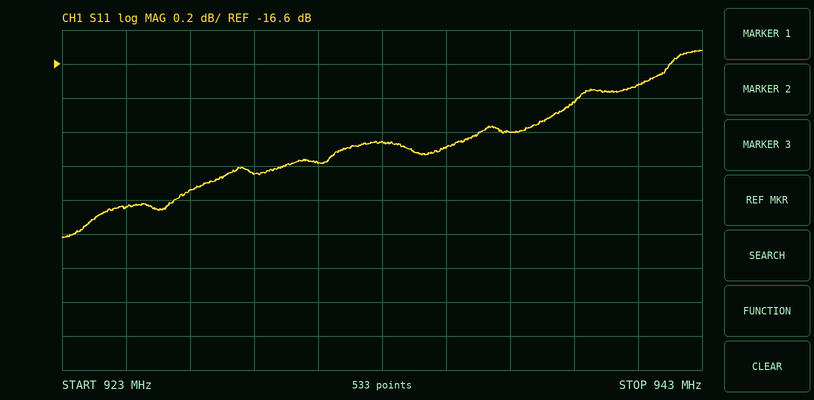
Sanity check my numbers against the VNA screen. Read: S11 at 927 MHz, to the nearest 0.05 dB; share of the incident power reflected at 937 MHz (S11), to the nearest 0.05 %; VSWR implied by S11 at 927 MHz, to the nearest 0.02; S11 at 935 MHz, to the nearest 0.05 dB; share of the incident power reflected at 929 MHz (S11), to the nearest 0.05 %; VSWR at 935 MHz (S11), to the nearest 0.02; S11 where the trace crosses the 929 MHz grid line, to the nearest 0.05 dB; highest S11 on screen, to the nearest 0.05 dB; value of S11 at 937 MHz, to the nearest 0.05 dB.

-17.35 dB
2.00 %
1.32
-17.10 dB
1.90 %
1.32
-17.25 dB
-16.50 dB
-17.00 dB
